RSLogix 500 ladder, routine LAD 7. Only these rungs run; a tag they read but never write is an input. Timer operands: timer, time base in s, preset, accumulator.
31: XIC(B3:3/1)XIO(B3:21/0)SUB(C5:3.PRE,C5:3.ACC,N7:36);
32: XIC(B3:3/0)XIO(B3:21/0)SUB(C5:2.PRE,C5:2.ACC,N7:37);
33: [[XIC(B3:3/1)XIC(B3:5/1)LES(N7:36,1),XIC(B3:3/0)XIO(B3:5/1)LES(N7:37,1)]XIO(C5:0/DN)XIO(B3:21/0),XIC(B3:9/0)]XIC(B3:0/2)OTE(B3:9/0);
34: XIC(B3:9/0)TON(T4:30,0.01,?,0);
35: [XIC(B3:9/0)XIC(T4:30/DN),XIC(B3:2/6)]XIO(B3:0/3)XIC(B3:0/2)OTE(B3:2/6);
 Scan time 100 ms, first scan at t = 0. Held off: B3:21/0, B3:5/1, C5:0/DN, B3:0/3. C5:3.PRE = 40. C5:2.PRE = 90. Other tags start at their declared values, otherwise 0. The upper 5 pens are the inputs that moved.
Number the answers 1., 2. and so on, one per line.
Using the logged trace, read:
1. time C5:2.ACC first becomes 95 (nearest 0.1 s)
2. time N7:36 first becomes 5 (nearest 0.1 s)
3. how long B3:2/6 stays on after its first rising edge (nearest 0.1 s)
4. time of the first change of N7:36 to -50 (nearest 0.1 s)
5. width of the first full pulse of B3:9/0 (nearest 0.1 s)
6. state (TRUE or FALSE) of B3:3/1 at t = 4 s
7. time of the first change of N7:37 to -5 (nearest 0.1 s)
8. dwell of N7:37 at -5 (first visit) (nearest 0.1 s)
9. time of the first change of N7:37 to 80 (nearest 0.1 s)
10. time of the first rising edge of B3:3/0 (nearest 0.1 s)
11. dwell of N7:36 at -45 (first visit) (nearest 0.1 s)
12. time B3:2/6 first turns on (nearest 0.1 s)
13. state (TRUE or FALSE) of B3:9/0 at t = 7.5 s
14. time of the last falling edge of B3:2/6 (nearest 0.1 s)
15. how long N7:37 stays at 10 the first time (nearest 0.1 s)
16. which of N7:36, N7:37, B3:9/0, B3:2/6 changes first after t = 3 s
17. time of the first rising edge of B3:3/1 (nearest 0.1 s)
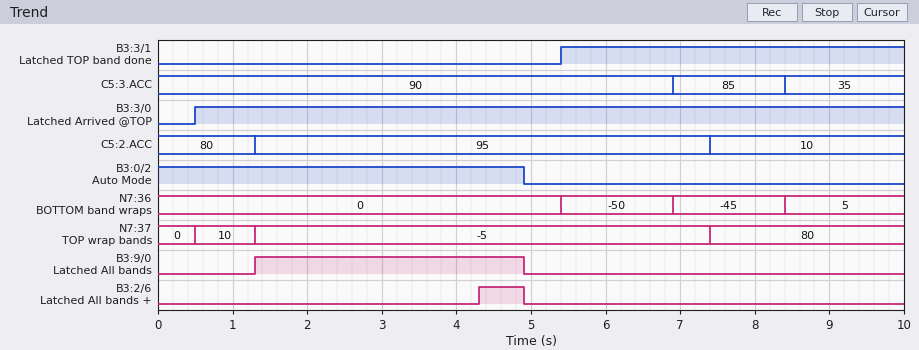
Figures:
1. 1.3 s
2. 8.4 s
3. 0.6 s
4. 5.4 s
5. 3.6 s
6. FALSE
7. 1.3 s
8. 6.1 s
9. 7.4 s
10. 0.5 s
11. 1.5 s
12. 4.3 s
13. FALSE
14. 4.9 s
15. 0.8 s
16. B3:2/6
17. 5.4 s
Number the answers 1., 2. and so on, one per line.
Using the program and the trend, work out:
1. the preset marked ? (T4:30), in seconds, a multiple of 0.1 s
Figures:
1. 3.0 s
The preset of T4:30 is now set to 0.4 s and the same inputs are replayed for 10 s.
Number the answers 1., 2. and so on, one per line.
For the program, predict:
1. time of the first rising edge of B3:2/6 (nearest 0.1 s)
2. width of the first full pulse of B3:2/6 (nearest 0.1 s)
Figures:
1. 1.7 s
2. 3.2 s
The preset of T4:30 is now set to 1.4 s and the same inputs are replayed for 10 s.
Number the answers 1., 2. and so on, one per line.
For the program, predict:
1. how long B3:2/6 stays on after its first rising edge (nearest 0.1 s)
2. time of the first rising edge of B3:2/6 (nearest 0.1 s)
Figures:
1. 2.2 s
2. 2.7 s
